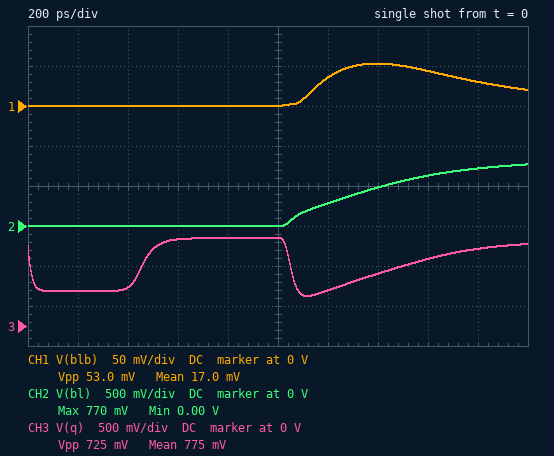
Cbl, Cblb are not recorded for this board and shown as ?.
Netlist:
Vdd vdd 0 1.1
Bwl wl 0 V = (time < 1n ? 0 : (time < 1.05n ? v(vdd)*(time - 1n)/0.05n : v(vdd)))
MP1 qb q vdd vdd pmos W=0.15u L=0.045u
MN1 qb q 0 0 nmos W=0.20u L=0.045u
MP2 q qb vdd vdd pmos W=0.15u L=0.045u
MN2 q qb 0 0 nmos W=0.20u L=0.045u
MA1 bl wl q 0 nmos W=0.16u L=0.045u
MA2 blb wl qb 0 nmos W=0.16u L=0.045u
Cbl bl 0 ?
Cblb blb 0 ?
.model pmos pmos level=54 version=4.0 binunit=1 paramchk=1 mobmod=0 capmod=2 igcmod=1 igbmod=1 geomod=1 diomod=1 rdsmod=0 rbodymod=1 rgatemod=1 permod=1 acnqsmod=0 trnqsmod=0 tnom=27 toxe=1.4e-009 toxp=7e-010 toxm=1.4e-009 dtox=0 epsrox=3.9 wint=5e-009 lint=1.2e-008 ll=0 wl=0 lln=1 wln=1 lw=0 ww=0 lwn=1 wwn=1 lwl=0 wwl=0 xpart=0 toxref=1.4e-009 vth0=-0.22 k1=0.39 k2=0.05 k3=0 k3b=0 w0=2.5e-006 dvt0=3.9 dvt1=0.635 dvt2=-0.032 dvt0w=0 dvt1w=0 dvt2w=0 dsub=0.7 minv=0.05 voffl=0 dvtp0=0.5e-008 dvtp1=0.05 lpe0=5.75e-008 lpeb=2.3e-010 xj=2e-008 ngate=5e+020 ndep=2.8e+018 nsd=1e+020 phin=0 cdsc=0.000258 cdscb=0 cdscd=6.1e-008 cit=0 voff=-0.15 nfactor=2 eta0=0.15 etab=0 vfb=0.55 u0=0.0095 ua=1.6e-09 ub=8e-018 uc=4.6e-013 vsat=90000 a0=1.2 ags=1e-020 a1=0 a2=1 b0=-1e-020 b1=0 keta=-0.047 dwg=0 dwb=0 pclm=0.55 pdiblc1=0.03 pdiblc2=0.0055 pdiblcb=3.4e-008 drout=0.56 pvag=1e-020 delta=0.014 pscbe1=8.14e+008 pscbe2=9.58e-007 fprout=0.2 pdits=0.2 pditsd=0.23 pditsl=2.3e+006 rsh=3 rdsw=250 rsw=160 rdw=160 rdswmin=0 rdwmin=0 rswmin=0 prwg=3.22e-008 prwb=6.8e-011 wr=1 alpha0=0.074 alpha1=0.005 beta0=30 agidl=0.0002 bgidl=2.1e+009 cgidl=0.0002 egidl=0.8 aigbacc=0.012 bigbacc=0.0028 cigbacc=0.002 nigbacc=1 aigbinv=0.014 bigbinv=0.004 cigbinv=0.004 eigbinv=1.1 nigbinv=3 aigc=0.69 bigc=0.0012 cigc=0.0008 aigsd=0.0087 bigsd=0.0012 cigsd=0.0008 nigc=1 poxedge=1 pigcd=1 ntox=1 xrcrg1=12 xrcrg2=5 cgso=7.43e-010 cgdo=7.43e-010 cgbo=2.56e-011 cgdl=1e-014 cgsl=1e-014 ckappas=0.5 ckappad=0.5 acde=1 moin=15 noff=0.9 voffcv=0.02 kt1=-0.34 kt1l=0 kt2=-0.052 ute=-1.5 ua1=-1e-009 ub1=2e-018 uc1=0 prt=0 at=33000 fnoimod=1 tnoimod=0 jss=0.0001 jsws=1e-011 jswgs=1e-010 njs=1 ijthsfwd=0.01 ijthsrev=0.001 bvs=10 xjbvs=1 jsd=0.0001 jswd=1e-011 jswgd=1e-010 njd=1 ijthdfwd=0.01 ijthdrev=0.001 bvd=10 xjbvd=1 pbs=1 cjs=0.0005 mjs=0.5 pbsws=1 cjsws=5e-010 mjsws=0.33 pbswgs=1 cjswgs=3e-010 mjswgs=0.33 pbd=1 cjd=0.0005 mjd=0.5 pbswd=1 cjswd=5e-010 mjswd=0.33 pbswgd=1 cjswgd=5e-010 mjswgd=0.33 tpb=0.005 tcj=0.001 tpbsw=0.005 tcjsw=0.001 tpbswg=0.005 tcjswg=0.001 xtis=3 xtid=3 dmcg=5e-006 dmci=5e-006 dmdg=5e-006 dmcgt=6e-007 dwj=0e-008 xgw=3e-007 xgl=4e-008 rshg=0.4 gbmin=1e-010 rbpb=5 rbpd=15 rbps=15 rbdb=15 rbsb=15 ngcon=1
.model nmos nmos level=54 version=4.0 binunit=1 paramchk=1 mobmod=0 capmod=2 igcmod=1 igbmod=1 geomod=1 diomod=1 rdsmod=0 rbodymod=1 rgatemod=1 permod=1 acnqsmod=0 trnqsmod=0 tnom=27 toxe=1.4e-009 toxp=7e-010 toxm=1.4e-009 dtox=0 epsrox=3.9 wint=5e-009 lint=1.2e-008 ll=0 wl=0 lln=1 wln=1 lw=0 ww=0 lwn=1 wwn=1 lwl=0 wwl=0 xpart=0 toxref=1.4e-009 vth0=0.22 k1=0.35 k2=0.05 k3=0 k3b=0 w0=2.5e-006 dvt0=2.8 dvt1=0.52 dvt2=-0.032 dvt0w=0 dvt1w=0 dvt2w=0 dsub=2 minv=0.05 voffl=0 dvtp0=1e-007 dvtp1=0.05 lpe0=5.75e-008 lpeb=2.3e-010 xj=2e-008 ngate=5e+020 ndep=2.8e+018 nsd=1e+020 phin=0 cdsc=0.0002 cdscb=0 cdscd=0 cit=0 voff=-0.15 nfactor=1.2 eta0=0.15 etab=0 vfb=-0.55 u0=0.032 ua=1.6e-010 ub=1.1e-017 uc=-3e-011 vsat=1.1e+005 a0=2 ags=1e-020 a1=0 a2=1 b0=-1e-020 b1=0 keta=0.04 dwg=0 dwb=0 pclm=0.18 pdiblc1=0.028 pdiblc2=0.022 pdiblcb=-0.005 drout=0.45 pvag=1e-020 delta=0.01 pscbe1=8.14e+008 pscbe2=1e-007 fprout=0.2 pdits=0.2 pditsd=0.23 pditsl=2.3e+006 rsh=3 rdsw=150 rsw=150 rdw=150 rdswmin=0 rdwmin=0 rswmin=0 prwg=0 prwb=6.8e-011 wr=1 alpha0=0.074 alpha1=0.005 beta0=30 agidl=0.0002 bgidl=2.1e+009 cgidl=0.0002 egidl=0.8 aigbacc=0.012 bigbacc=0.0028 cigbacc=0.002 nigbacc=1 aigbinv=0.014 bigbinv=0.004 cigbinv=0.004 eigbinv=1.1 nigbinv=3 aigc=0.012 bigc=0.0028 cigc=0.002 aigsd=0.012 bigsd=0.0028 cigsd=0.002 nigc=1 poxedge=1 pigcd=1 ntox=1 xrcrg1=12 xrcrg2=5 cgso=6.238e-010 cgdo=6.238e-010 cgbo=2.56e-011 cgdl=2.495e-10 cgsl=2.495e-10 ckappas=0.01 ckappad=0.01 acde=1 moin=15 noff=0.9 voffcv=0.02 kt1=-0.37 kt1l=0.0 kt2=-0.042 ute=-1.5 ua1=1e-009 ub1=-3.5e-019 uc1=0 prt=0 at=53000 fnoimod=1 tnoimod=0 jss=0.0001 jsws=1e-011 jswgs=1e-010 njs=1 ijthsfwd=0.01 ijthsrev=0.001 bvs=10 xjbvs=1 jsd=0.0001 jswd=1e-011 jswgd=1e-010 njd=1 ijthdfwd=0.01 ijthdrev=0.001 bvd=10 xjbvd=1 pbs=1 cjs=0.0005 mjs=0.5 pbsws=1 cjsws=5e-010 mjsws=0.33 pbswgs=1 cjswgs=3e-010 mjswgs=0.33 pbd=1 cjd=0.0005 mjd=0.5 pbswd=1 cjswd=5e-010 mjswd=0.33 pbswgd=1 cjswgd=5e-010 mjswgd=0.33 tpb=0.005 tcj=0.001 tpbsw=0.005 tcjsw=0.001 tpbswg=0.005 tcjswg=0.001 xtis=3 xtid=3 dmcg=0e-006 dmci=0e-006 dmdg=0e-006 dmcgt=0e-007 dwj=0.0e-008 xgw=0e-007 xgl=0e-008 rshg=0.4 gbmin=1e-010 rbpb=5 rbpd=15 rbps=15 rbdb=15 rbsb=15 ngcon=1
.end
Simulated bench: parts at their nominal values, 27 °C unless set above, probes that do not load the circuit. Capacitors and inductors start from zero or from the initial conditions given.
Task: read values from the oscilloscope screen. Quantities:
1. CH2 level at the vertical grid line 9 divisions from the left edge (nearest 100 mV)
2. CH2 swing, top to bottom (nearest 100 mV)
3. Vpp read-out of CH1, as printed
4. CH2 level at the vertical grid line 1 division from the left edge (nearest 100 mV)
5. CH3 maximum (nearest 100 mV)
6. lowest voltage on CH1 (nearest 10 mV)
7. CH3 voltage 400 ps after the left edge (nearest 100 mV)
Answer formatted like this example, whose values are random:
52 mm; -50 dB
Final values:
700 mV; 800 mV; 53.0 mV; 0 V; 1.1 V; 0 V; 500 mV
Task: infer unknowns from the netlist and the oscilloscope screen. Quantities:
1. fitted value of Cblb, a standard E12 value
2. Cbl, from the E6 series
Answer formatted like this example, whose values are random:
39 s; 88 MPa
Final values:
100 fF; 47 fF
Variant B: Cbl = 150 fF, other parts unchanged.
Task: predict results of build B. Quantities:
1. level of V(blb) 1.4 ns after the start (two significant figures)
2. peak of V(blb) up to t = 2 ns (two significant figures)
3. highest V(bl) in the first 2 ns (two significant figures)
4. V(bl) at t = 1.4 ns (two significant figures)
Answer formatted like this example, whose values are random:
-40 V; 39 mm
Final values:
250 mV; 530 mV; 97 mV; 80 mV
